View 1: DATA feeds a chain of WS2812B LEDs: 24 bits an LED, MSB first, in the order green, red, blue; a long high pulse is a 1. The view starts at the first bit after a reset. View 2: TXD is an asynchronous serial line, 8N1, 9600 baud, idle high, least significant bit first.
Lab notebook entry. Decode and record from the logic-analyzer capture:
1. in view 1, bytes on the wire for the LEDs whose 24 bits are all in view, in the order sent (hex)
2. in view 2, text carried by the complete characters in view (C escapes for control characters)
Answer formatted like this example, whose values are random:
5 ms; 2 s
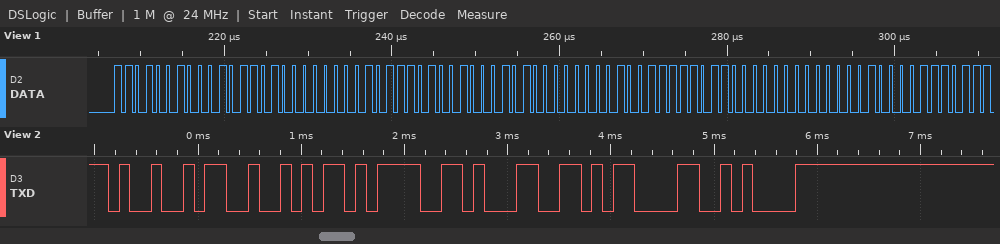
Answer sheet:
D2 2D 00 BA 45 00 9F 60 00; "IR=1\r\n"
